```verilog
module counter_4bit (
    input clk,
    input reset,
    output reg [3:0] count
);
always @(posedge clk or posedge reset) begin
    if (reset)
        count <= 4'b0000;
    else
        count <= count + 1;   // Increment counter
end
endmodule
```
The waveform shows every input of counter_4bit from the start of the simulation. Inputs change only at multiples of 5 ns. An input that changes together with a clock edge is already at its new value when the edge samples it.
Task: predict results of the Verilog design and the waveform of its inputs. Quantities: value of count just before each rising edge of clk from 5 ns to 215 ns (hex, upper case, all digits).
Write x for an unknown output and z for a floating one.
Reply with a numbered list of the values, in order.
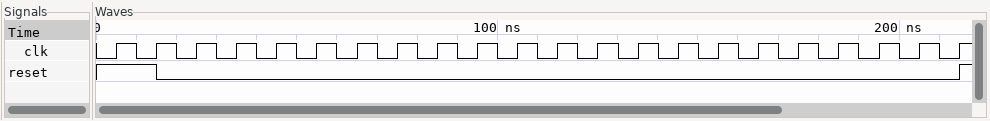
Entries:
1. 0, 0, 1, 2, 3, 4, 5, 6, 7, 8, 9, A, B, C, D, E, F, 0, 1, 2, 3, 4
